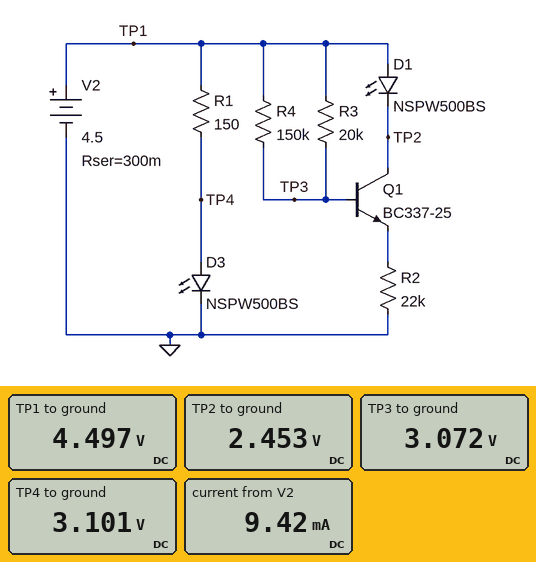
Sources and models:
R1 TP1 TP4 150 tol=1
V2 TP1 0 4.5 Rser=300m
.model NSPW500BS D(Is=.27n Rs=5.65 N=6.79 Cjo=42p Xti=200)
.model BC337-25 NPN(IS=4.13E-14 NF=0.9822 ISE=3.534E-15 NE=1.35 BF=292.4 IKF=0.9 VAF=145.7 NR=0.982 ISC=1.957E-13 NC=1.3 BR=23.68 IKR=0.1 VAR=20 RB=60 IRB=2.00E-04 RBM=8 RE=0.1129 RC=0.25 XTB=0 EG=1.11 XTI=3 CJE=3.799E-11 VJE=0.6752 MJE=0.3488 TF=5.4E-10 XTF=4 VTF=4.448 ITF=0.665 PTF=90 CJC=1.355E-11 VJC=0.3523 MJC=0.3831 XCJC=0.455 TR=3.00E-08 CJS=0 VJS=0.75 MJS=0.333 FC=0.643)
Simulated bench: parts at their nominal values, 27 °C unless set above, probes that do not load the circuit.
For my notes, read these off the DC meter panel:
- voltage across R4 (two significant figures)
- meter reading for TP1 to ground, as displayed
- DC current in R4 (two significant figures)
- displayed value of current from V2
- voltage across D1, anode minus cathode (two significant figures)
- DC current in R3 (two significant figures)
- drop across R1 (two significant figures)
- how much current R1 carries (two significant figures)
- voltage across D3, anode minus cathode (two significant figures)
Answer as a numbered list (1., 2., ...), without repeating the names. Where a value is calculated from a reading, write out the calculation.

1. 4.497 V - 3.072 V = 1.4 V
2. 4.497 V
3. (4.497 V - 3.072 V) / 150 kΩ = 9.5 µA
4. 9.42 mA
5. 4.497 V - 2.453 V = 2.0 V
6. (4.497 V - 3.072 V) / 20 kΩ = 71 µA
7. 4.497 V - 3.101 V = 1.4 V
8. (4.497 V - 3.101 V) / 150 Ω = 9.3 mA
9. 3.101 V = 3.1 V
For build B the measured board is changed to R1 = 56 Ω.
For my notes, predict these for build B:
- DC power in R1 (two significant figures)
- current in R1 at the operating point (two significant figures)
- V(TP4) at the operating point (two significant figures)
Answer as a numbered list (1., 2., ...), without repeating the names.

1. 25 mW
2. 21 mA
3. 3.3 V
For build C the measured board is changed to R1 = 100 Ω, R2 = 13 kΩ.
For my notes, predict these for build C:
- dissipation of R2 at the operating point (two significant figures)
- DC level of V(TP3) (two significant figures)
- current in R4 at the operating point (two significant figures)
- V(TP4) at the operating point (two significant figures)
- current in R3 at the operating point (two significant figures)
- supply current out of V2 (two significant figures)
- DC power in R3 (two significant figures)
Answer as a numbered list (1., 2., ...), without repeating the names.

1. 400 µW
2. 2.9 V
3. 11 µA
4. 3.2 V
5. 80 µA
6. 13 mA
7. 130 µW
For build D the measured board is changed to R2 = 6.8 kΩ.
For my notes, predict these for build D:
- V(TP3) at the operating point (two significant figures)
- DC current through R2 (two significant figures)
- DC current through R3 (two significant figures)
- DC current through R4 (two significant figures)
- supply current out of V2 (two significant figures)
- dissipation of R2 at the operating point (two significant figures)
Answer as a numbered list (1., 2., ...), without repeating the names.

1. 2.7 V
2. 310 µA
3. 88 µA
4. 12 µA
5. 9.6 mA
6. 650 µW
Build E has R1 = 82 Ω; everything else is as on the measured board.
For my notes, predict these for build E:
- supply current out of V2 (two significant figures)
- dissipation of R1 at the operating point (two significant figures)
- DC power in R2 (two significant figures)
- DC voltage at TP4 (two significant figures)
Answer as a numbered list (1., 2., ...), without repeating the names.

1. 16 mA
2. 20 mW
3. 270 µW
4. 3.2 V
